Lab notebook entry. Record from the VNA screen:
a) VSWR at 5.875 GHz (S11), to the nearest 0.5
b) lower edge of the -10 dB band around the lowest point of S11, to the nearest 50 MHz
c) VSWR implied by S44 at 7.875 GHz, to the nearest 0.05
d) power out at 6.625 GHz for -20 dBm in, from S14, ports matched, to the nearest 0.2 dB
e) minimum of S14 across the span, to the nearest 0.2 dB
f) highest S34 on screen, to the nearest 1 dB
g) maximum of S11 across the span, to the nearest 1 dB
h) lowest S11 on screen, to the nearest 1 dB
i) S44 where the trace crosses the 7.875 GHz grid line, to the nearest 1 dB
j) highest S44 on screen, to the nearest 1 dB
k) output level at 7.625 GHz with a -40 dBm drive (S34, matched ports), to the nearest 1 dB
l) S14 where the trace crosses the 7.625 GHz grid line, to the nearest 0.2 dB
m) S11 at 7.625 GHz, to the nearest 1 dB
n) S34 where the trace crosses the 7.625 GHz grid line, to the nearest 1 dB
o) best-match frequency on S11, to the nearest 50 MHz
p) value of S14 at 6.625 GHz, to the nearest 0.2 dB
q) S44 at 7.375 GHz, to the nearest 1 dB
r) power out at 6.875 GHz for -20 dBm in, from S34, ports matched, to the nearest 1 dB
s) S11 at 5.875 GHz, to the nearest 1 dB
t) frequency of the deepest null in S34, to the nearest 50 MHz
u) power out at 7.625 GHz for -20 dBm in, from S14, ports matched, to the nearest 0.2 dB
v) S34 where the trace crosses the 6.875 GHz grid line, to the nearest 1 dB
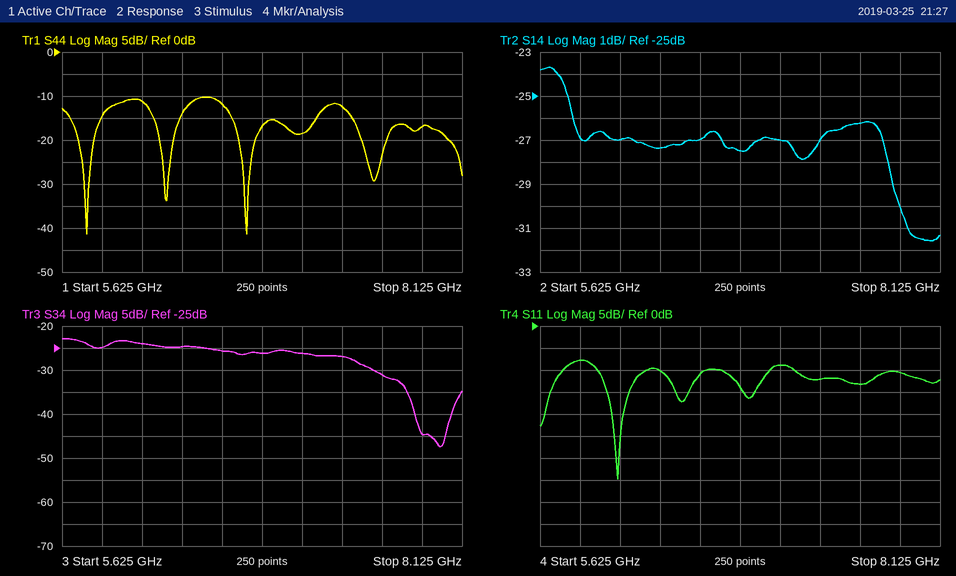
2.5
6.00 GHz
1.35
-47.0 dBm
-31.6 dB
-23 dB
-8 dB
-35 dB
-17 dB
-10 dB
-71 dBm
-26.2 dB
-13 dB
-31 dB
6.10 GHz
-27.0 dB
-12 dB
-46 dBm
-8 dB
8.00 GHz
-46.2 dBm
-26 dB
